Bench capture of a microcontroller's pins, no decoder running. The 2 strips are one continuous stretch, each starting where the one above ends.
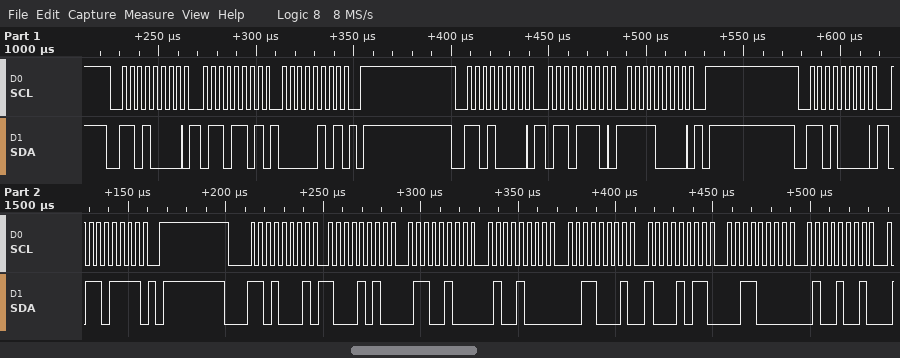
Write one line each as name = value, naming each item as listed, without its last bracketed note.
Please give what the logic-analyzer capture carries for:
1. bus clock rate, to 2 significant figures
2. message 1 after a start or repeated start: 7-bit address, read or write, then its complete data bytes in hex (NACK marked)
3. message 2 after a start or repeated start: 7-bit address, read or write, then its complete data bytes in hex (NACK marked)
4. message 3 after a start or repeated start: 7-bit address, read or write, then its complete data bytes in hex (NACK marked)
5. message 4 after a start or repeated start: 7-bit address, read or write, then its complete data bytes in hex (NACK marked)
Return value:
bus clock rate, to 2 significant figures = 250 kHz
message 1 after a start or repeated start: 7-bit address, read or write, then its complete data bytes in hex = 0x68 write: 6D 05
message 2 after a start or repeated start: 7-bit address, read or write, then its complete data bytes in hex = 0x68 write: 6E F0
message 3 after a start or repeated start: 7-bit address, read or write, then its complete data bytes in hex = 0x68 write: 6F
message 4 after a start or repeated start: 7-bit address, read or write, then its complete data bytes in hex = 0x68 read: 8A 64 48 31 8B 30 49
